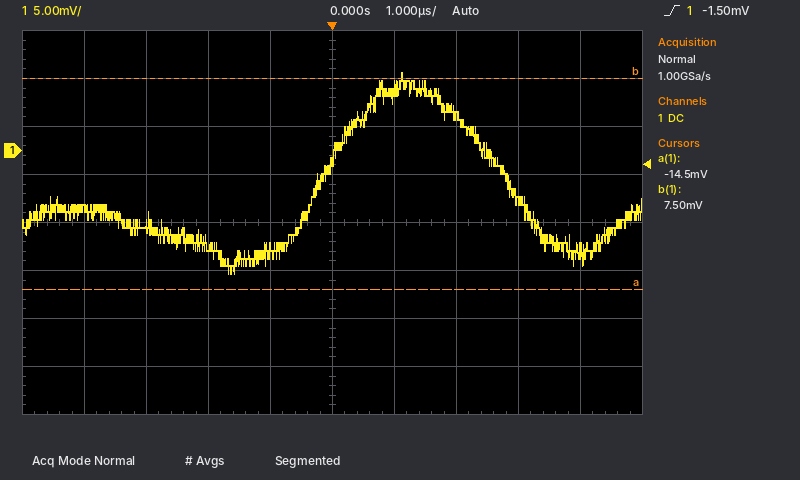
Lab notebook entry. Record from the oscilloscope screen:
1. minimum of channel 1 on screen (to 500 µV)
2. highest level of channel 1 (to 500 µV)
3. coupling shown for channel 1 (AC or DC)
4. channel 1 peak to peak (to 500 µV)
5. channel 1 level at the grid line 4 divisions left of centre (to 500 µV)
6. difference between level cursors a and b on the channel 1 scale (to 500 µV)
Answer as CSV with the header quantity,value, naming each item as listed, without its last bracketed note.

quantity,value
minimum of channel 1 on screen,-13.0 mV
highest level of channel 1,8.0 mV
coupling shown for channel 1,DC
channel 1 peak to peak,21.0 mV
channel 1 level at the grid line 4 divisions left of centre,-6.0 mV
difference between level cursors a and b on the channel 1 scale,22.0 mV
